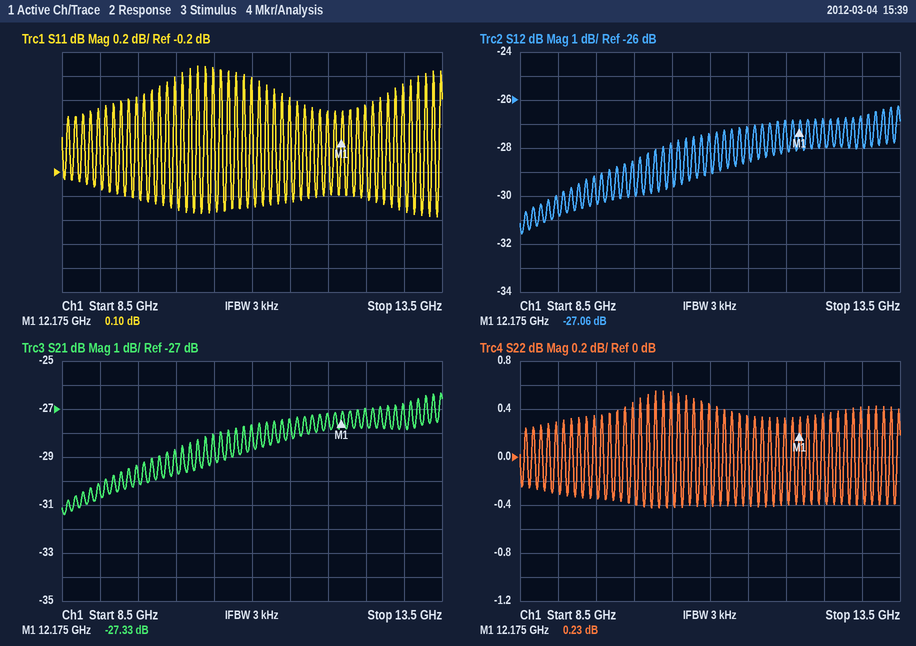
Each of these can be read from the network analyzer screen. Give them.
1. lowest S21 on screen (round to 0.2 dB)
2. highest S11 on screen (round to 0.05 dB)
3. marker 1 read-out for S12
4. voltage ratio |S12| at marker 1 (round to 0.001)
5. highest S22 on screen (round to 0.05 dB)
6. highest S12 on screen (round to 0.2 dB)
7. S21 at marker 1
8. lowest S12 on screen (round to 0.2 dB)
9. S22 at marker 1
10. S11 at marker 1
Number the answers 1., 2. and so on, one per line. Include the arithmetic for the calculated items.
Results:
1. -31.4 dB
2. 0.70 dB
3. -27.06 dB
4. 10^(-27.06/20) ≈ 0.044
5. 0.55 dB
6. -26.2 dB
7. -27.33 dB
8. -31.6 dB
9. 0.23 dB
10. 0.10 dB
